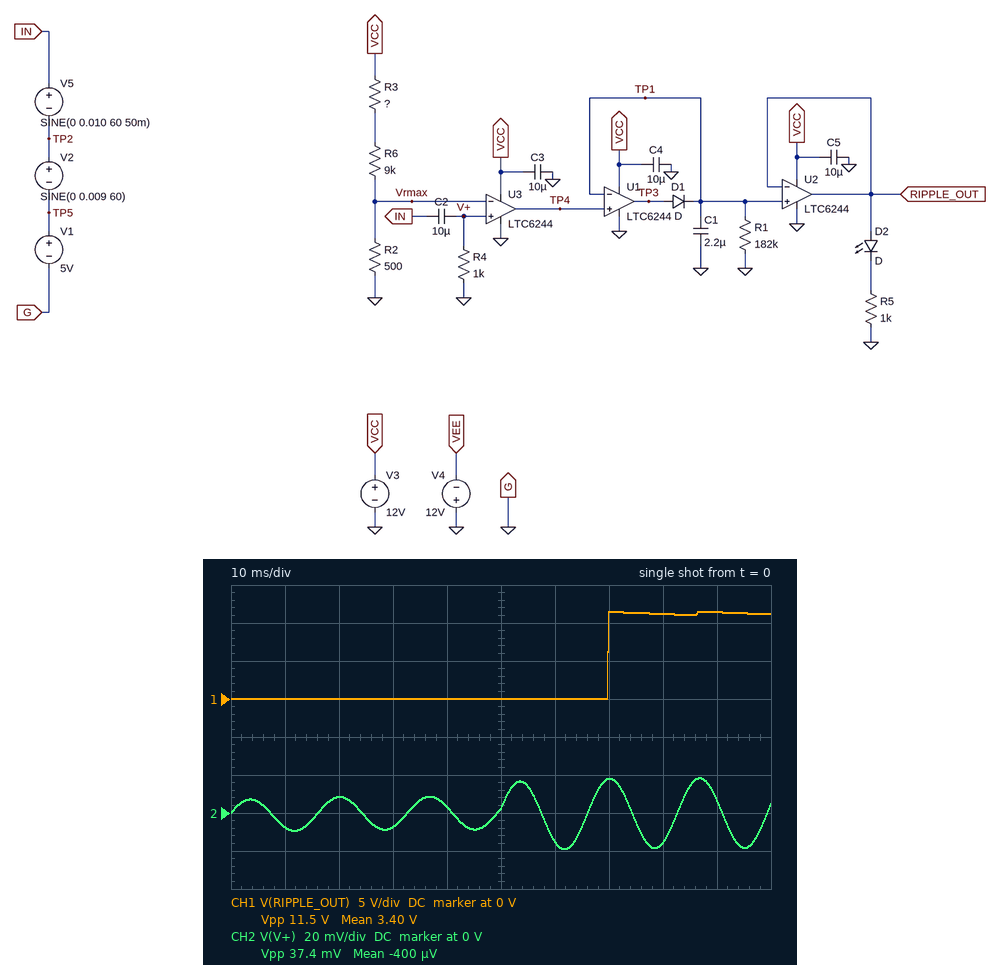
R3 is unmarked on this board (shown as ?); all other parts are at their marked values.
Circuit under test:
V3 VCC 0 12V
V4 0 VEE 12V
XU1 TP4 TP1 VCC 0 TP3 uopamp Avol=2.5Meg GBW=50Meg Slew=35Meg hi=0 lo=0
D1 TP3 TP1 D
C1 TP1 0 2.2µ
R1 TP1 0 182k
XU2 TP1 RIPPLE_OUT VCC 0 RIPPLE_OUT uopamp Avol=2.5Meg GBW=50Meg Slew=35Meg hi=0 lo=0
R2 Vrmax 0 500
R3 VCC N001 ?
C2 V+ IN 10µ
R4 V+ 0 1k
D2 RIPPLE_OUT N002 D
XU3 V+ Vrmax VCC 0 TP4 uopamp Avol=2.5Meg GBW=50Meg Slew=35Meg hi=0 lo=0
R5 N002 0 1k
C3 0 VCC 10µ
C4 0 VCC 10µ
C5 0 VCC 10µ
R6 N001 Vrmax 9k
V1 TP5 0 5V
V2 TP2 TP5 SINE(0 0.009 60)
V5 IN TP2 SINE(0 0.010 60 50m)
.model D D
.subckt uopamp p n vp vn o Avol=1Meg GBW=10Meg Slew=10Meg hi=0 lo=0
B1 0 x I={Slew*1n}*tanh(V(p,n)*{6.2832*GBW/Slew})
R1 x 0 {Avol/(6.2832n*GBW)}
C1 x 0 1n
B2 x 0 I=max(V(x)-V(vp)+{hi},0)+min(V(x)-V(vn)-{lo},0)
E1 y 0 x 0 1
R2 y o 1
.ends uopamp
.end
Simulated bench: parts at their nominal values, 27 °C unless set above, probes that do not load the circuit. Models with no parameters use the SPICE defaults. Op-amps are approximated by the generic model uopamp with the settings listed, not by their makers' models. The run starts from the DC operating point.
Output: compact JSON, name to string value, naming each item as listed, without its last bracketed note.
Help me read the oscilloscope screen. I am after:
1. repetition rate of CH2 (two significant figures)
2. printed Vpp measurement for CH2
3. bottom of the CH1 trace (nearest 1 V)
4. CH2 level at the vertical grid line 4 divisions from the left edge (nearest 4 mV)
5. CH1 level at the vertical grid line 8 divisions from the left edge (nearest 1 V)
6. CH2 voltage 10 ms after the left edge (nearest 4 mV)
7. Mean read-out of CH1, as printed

{"repetition rate of CH2": "60 Hz", "printed Vpp measurement for CH2": "37.4 mV", "bottom of the CH1 trace": "0 V", "CH2 level at the vertical grid line 4 divisions from the left edge": "4 mV", "CH1 level at the vertical grid line 8 divisions from the left edge": "11 V", "CH2 voltage 10 ms after the left edge": "-8 mV", "Mean read-out of CH1, as printed": "3.40 V"}
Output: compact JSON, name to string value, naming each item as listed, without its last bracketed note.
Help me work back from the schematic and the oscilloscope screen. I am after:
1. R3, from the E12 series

{"R3, from the E12 series": "330 kΩ"}
